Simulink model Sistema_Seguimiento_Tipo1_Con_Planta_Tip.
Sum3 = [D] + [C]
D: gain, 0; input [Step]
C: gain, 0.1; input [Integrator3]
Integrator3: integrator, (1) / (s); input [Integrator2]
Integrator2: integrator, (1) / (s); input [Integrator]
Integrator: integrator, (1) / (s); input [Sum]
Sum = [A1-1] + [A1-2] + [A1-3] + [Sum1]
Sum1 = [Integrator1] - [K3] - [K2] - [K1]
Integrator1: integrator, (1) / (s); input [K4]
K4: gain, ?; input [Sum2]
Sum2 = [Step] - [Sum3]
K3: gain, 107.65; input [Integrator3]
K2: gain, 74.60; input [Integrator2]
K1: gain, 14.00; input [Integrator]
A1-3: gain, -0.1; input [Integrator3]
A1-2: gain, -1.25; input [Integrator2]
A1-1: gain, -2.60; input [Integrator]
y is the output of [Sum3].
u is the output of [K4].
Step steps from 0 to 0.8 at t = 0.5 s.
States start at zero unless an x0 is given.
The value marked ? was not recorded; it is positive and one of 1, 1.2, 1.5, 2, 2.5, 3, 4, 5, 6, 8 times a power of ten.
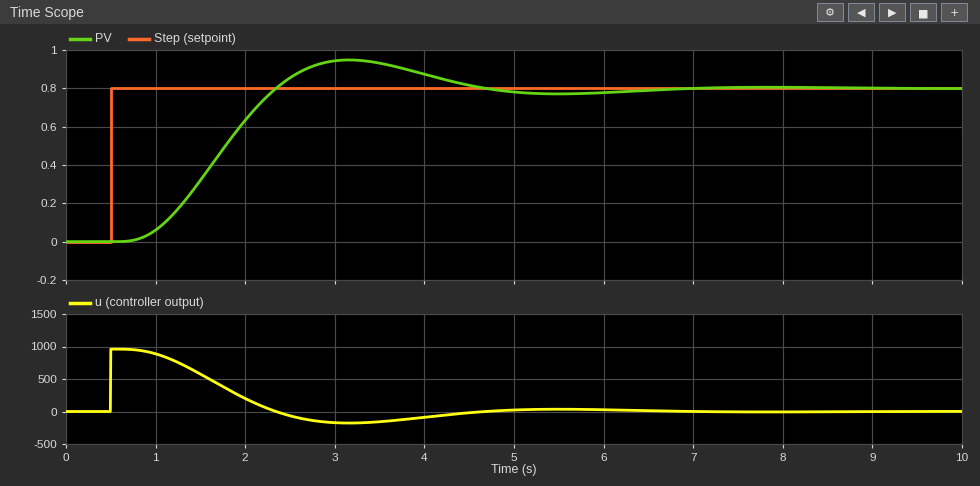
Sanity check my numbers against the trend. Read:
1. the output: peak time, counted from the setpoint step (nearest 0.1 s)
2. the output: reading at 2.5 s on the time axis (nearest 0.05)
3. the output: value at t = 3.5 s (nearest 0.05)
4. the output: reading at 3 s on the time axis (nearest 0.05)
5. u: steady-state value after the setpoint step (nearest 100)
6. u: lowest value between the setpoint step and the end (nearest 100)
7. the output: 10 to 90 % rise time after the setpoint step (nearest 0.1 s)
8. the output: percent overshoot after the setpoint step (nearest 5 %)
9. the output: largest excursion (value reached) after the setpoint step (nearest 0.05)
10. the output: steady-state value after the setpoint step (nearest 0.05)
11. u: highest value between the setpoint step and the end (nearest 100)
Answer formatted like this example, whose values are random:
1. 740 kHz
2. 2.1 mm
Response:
1. 2.7 s
2. 0.85
3. 0.95
4. 0.95
5. 0
6. -200
7. 1.1 s
8. 20 %
9. 0.95
10. 0.80
11. 1000
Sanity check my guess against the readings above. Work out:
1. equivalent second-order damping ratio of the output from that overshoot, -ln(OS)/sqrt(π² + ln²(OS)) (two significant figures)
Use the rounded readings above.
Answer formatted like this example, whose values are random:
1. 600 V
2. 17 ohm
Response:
1. 0.46
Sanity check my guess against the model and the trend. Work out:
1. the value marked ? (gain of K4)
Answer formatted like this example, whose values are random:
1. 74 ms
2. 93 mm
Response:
1. 1200
